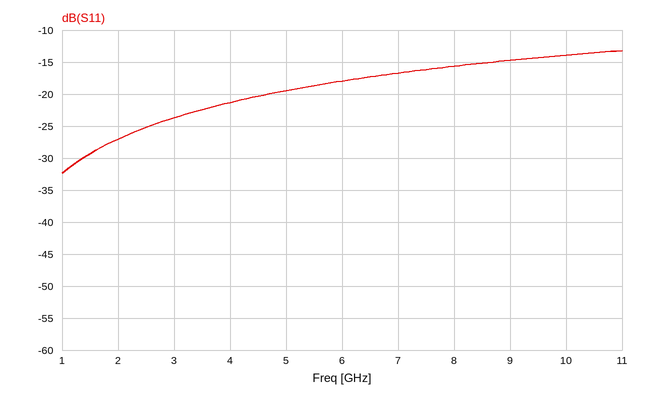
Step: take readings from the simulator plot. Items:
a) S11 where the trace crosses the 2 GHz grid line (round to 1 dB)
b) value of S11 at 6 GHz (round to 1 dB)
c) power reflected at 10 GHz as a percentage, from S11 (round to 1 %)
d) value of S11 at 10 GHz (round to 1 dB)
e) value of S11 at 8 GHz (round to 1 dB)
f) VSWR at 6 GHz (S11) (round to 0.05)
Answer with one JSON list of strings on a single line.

["-27 dB", "-18 dB", "4 %", "-14 dB", "-16 dB", "1.30"]
